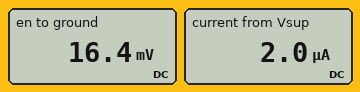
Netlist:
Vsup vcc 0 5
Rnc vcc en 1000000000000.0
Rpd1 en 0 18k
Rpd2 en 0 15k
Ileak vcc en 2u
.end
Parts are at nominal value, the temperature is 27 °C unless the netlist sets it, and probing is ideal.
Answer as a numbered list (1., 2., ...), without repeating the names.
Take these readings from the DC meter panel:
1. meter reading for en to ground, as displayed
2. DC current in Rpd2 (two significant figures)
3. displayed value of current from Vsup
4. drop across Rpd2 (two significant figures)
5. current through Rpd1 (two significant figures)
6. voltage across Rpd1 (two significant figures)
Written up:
1. 16.4 mV
2. 1.1 µA
3. 2.0 µA
4. 16 mV
5. 910 nA
6. 16 mV
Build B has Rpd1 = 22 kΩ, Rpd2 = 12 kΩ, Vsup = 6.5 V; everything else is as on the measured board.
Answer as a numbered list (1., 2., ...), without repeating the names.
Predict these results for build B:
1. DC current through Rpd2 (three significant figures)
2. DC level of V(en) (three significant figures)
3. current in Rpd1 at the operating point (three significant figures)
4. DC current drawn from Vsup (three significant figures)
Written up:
1. 1.29 µA
2. 15.5 mV
3. 706 nA
4. 2.00 µA
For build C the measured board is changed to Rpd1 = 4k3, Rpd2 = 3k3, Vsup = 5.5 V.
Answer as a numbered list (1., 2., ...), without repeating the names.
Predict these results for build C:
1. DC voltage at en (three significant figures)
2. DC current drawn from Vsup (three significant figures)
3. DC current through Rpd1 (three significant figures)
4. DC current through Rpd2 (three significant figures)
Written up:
1. 3.73 mV
2. 2.00 µA
3. 868 nA
4. 1.13 µA
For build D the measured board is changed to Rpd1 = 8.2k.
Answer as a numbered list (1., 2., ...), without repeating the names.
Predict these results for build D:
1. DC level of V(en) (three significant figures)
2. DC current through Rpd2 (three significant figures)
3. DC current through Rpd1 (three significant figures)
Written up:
1. 10.6 mV
2. 707 nA
3. 1.29 µA
